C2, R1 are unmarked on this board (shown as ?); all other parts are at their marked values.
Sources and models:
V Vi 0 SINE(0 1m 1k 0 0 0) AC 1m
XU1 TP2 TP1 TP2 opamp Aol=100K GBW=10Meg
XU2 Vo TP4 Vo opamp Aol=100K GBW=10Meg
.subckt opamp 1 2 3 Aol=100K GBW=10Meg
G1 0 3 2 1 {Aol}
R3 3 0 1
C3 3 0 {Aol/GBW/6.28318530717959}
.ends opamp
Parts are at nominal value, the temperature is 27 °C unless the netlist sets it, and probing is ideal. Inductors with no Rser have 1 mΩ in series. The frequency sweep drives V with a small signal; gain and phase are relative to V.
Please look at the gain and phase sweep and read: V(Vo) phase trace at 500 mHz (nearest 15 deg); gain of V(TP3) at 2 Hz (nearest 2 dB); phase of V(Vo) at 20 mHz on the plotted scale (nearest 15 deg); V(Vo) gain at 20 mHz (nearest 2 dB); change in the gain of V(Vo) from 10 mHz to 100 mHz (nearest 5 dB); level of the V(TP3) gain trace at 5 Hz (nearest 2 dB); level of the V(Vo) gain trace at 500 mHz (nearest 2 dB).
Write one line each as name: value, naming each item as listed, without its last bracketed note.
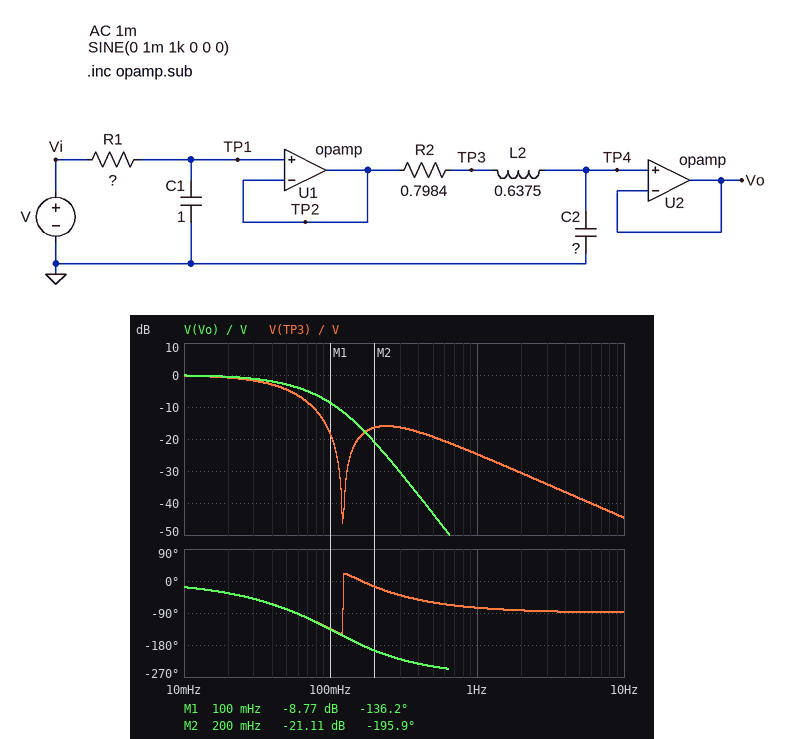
V(Vo) phase trace at 500 mHz: -240 deg
gain of V(TP3) at 2 Hz: -30 dB
phase of V(Vo) at 20 mHz on the plotted scale: -30 deg
V(Vo) gain at 20 mHz: 0 dB
change in the gain of V(Vo) from 10 mHz to 100 mHz: -10 dB
level of the V(TP3) gain trace at 5 Hz: -38 dB
level of the V(Vo) gain trace at 500 mHz: -44 dB
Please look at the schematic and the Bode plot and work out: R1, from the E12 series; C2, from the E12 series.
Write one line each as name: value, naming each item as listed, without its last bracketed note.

R1, from the E12 series: 2.7 Ω
C2, from the E12 series: 2.7 F
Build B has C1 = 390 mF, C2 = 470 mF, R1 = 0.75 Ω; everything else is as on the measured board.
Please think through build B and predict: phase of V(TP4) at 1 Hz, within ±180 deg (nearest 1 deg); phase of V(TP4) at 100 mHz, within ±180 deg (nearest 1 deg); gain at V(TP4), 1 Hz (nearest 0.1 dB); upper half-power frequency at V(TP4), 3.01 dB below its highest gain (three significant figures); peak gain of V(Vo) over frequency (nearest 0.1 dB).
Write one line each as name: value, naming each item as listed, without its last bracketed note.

phase of V(TP4) at 1 Hz, within ±180 deg: 131 deg
phase of V(TP4) at 100 mHz, within ±180 deg: -25 deg
gain at V(TP4), 1 Hz: -27.3 dB
upper half-power frequency at V(TP4), 3.01 dB below its highest gain: 335 mHz
peak gain of V(Vo) over frequency: 3.0 dB
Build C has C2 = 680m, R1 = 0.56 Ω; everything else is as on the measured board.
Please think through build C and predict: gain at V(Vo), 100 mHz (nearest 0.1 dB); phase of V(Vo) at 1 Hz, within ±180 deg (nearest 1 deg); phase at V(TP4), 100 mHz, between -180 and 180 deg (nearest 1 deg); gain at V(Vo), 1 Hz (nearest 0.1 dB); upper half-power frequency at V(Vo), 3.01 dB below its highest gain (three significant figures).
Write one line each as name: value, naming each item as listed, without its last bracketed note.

gain at V(Vo), 100 mHz: 0.4 dB
phase of V(Vo) at 1 Hz, within ±180 deg: 118 deg
phase at V(TP4), 100 mHz, between -180 and 180 deg: -42 deg
gain at V(Vo), 1 Hz: -35.6 dB
upper half-power frequency at V(Vo), 3.01 dB below its highest gain: 265 mHz
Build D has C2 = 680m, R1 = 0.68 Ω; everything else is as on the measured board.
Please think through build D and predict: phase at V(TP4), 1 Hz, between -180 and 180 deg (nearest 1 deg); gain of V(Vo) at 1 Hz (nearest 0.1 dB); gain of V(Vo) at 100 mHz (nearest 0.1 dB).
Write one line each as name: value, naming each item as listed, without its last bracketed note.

phase at V(TP4), 1 Hz, between -180 and 180 deg: 115 deg
gain of V(Vo) at 1 Hz: -37.2 dB
gain of V(Vo) at 100 mHz: 0.2 dB
